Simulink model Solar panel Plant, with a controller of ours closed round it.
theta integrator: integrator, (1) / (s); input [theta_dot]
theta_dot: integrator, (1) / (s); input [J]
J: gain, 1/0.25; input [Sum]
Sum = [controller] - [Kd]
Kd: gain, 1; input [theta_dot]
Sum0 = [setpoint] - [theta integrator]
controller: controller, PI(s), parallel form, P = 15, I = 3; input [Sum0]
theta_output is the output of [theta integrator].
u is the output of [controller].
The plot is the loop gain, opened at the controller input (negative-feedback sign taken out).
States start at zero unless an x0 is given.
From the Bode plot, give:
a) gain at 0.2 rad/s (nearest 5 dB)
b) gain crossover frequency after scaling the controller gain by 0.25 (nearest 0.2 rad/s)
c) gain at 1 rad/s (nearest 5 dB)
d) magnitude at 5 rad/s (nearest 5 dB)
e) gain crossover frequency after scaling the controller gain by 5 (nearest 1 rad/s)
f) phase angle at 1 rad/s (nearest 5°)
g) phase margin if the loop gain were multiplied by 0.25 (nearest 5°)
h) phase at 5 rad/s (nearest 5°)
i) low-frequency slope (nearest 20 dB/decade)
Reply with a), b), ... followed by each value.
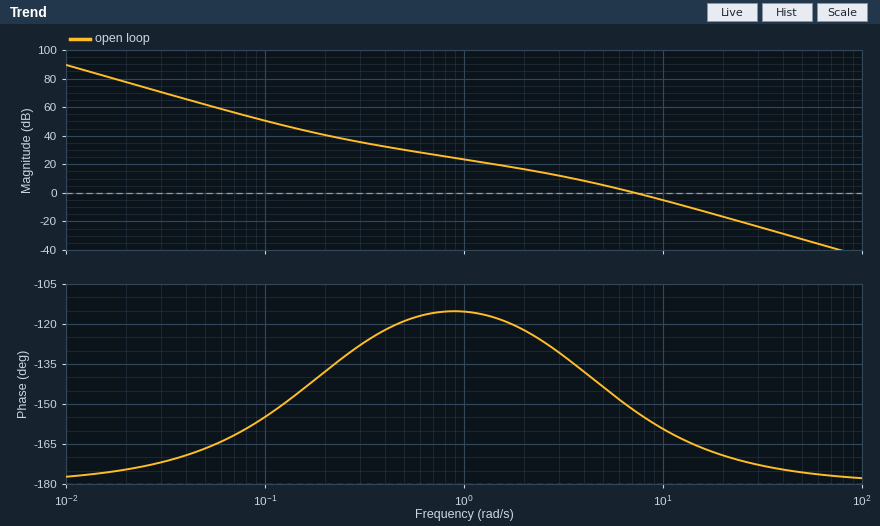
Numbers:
a) 40 dB
b) 3.0 rad/s
c) 25 dB
d) 5 dB
e) 17 rad/s
f) -115°
g) 50°
h) -145°
i) -40 dB/decade
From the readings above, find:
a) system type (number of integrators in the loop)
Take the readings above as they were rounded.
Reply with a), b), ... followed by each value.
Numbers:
a) 2
